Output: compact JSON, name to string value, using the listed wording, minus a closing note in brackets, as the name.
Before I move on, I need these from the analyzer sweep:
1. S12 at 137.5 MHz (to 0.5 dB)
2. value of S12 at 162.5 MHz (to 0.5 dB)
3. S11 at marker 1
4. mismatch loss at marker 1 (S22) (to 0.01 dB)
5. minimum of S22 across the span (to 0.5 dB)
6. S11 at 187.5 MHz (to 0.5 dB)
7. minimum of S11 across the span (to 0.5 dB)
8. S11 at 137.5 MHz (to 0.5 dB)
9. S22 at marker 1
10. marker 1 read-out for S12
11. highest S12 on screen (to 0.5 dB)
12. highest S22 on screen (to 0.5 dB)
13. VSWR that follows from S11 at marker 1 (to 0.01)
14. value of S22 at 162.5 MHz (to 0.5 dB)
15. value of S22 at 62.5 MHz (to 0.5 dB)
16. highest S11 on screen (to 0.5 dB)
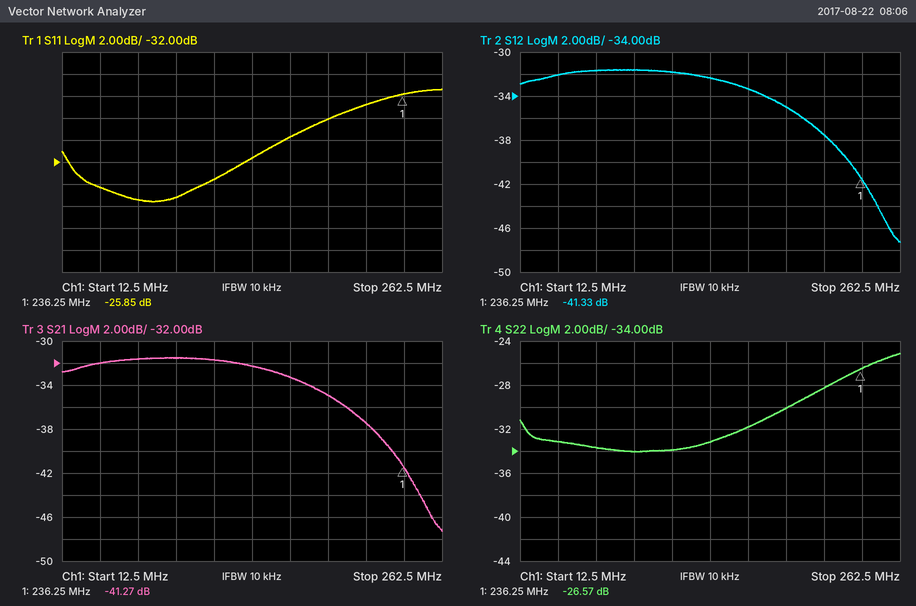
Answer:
{"S12 at 137.5 MHz": "-32.5 dB", "value of S12 at 162.5 MHz": "-33.5 dB", "S11 at marker 1": "-25.85 dB", "mismatch loss at marker 1 (S22)": "0.01 dB", "minimum of S22 across the span": "-34.0 dB", "S11 at 187.5 MHz": "-28.0 dB", "minimum of S11 across the span": "-35.5 dB", "S11 at 137.5 MHz": "-31.5 dB", "S22 at marker 1": "-26.57 dB", "marker 1 read-out for S12": "-41.33 dB", "highest S12 on screen": "-31.5 dB", "highest S22 on screen": "-25.0 dB", "VSWR that follows from S11 at marker 1": "1.11", "value of S22 at 162.5 MHz": "-32.0 dB", "value of S22 at 62.5 MHz": "-33.5 dB", "highest S11 on screen": "-25.5 dB"}
